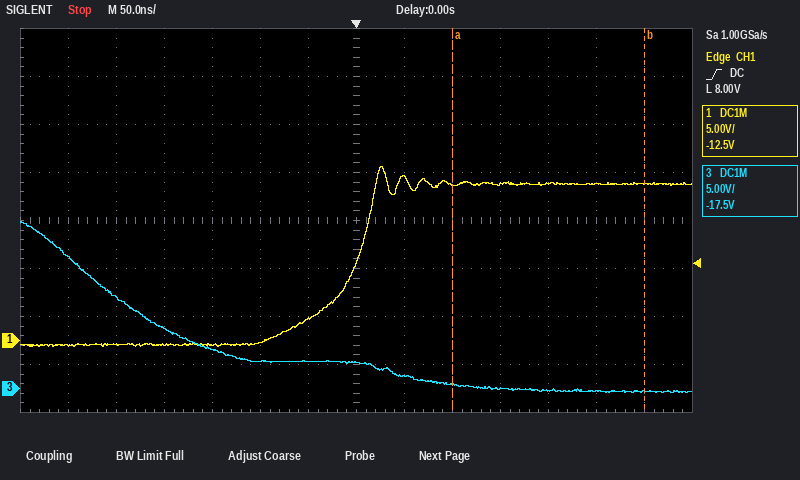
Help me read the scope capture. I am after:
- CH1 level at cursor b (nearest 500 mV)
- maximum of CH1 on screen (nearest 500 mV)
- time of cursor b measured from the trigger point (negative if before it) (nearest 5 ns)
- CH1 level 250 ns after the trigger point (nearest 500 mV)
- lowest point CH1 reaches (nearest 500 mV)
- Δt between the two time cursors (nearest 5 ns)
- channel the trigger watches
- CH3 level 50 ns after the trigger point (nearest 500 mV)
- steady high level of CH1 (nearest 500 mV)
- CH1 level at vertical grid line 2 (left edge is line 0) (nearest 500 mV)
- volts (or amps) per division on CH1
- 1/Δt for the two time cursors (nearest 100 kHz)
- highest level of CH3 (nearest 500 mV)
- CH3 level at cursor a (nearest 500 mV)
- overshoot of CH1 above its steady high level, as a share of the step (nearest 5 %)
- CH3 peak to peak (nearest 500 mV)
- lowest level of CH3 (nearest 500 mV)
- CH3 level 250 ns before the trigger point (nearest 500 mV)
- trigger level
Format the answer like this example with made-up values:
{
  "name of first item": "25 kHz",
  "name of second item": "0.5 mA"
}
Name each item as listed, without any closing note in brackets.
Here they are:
{
  "CH1 level at cursor b": "16.5 V",
  "maximum of CH1 on screen": "18.0 V",
  "time of cursor b measured from the trigger point (negative if before it)": "+300 ns",
  "CH1 level 250 ns after the trigger point": "16.5 V",
  "lowest point CH1 reaches": "-500 mV",
  "Δt between the two time cursors": "200 ns",
  "channel the trigger watches": "CH1",
  "CH3 level 50 ns after the trigger point": "1.5 V",
  "steady high level of CH1": "16.5 V",
  "CH1 level at vertical grid line 2 (left edge is line 0)": "-500 mV",
  "volts (or amps) per division on CH1": "5 V",
  "1/Δt for the two time cursors": "5.0 MHz",
  "highest level of CH3": "17.5 V",
  "CH3 level at cursor a": "500 mV",
  "overshoot of CH1 above its steady high level, as a share of the step": "10 %",
  "CH3 peak to peak": "18.0 V",
  "lowest level of CH3": "-500 mV",
  "CH3 level 250 ns before the trigger point": "9.5 V",
  "trigger level": "8.00 V"
}
